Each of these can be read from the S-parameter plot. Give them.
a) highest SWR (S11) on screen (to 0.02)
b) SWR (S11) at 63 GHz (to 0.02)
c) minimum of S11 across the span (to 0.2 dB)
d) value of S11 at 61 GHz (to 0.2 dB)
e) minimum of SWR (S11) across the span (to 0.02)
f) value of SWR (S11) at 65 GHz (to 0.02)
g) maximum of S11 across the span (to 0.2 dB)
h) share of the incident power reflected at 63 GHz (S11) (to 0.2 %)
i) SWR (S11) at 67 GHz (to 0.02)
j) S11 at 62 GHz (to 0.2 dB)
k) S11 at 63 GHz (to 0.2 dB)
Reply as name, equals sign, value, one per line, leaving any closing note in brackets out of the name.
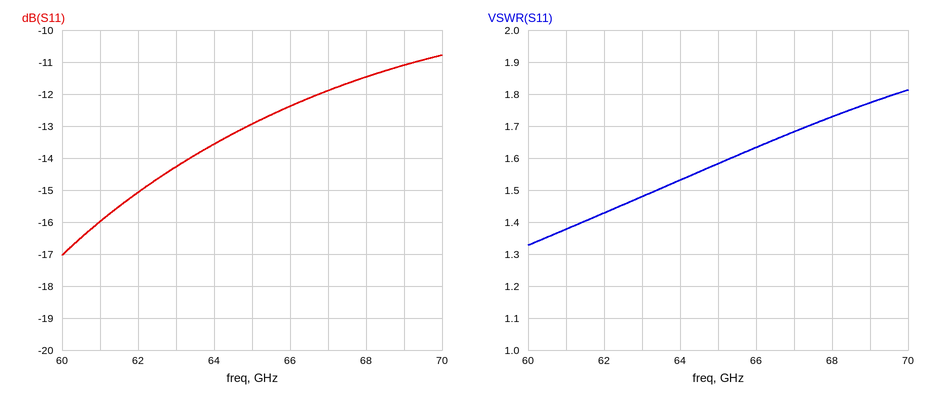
highest SWR (S11) on screen = 1.82
SWR (S11) at 63 GHz = 1.48
minimum of S11 across the span = -17.0 dB
value of S11 at 61 GHz = -16.0 dB
minimum of SWR (S11) across the span = 1.32
value of SWR (S11) at 65 GHz = 1.58
maximum of S11 across the span = -10.8 dB
share of the incident power reflected at 63 GHz (S11) = 3.8 %
SWR (S11) at 67 GHz = 1.68
S11 at 62 GHz = -15.0 dB
S11 at 63 GHz = -14.2 dB
